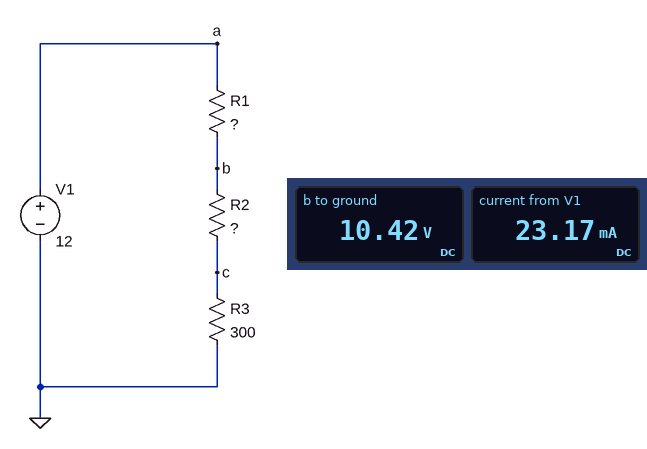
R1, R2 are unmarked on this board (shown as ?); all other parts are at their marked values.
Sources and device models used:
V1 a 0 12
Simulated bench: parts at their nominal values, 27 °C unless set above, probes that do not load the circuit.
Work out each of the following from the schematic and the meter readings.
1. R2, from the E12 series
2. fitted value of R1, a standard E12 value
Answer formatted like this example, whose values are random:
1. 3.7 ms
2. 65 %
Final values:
1. 150 Ω
2. 68 Ω
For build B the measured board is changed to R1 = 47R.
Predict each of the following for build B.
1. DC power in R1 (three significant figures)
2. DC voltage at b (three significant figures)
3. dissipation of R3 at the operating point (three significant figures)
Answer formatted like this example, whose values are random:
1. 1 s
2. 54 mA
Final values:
1. 27.4 mW
2. 10.9 V
3. 175 mW
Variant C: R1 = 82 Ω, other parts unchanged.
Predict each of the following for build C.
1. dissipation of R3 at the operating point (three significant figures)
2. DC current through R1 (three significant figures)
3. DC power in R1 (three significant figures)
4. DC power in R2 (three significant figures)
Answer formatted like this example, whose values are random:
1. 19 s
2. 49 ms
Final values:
1. 153 mW
2. 22.6 mA
3. 41.7 mW
4. 76.3 mW
